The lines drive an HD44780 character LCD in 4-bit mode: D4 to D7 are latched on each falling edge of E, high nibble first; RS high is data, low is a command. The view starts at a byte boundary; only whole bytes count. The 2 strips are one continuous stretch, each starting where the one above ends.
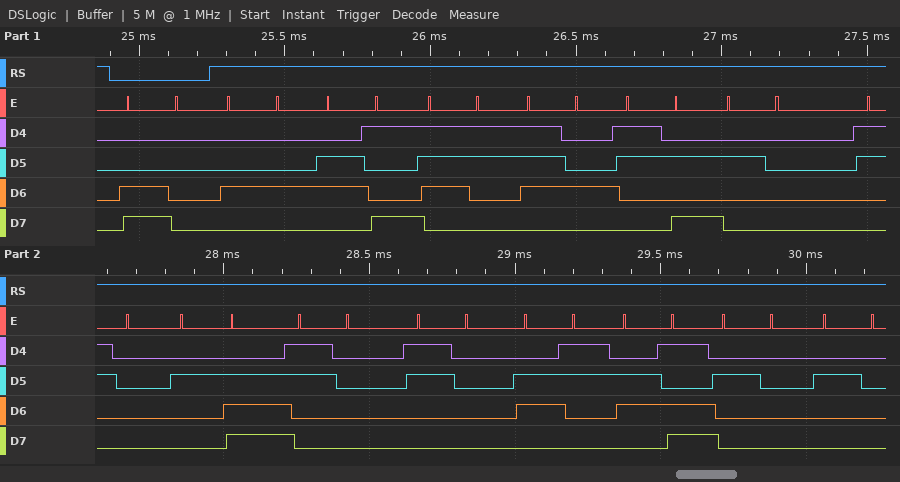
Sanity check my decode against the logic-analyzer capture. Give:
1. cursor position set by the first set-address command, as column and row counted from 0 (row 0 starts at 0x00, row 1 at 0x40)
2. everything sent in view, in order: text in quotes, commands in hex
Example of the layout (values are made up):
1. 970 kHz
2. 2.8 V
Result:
1. column 0, row 1
2. 0xC0 "Dist: 0.00cm  "
